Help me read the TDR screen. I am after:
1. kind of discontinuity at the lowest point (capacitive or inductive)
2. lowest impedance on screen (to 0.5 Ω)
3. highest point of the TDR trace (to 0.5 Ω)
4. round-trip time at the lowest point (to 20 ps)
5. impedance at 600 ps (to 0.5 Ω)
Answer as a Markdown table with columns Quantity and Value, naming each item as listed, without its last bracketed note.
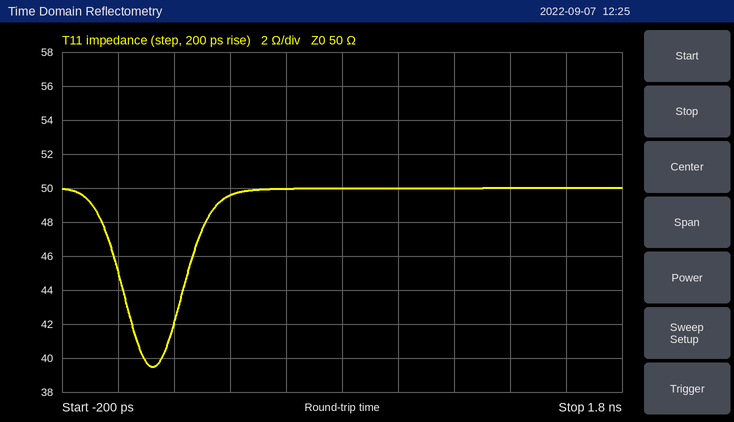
| Quantity | Value |
|---|---|
| kind of discontinuity at the lowest point | capacitive |
| lowest impedance on screen | 39.5 Ω |
| highest point of the TDR trace | 50.0 Ω |
| round-trip time at the lowest point | 120 ps |
| impedance at 600 ps | 50.0 Ω |
